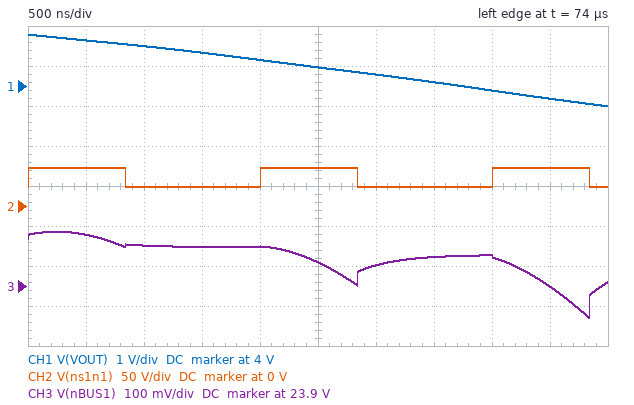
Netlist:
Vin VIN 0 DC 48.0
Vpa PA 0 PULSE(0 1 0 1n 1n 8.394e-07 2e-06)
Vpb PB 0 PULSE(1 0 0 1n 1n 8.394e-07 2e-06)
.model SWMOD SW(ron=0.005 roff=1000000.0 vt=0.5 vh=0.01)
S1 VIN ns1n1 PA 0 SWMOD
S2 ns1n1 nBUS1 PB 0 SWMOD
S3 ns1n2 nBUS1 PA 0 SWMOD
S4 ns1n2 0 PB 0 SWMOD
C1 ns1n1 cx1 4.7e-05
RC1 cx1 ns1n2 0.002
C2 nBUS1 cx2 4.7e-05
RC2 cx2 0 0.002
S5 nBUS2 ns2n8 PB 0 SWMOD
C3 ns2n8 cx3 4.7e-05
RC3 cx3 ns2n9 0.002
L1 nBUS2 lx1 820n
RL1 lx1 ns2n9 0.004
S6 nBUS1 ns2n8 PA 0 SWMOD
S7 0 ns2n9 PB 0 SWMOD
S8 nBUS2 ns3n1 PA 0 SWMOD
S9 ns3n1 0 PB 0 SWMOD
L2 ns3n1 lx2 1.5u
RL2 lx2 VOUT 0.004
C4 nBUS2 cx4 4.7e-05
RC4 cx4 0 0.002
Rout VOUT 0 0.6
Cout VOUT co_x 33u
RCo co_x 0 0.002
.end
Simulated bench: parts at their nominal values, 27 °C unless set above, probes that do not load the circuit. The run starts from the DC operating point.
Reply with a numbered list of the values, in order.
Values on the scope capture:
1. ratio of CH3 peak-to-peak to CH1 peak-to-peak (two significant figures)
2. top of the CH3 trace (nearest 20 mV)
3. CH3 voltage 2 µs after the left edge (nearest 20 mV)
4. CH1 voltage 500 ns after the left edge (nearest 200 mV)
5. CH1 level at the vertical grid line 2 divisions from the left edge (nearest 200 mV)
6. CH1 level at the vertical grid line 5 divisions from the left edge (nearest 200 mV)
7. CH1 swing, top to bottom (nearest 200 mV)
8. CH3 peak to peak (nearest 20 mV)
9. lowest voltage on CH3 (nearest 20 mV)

1. 0.12
2. 24.04 V
3. 24.00 V
4. 5.2 V
5. 5.0 V
6. 4.4 V
7. 1.8 V
8. 220 mV
9. 23.82 V
